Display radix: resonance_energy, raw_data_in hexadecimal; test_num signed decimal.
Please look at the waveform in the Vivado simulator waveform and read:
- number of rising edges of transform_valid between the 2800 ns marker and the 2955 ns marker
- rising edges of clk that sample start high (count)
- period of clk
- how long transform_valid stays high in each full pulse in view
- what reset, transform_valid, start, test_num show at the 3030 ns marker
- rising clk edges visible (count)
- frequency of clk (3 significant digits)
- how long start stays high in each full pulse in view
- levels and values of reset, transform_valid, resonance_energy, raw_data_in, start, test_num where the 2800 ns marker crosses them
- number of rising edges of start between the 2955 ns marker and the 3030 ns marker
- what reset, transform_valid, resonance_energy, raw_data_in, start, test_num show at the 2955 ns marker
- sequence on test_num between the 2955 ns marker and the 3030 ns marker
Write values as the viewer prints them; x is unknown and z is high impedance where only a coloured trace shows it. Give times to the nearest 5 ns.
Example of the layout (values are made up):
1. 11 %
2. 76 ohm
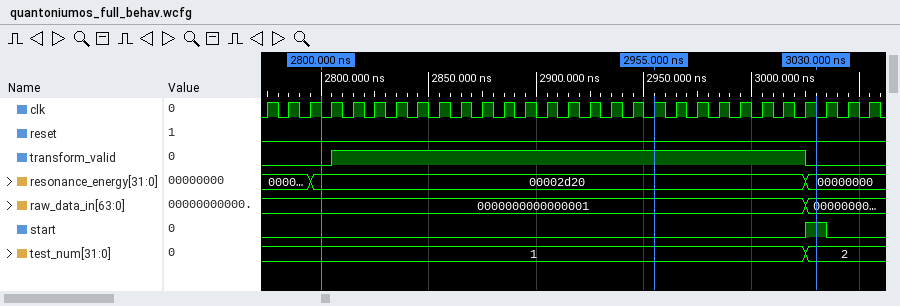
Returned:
1. 1
2. 1
3. 10 ns
4. 220 ns
5. reset=0, transform_valid=0, start=1, test_num=2
6. 29
7. 100 MHz
8. 10 ns
9. reset=0, transform_valid=0, resonance_energy=00002d20, raw_data_in=0000000000000001, start=0, test_num=1
10. 1
11. reset=0, transform_valid=1, resonance_energy=00002d20, raw_data_in=0000000000000001, start=0, test_num=1
12. 1, 2
